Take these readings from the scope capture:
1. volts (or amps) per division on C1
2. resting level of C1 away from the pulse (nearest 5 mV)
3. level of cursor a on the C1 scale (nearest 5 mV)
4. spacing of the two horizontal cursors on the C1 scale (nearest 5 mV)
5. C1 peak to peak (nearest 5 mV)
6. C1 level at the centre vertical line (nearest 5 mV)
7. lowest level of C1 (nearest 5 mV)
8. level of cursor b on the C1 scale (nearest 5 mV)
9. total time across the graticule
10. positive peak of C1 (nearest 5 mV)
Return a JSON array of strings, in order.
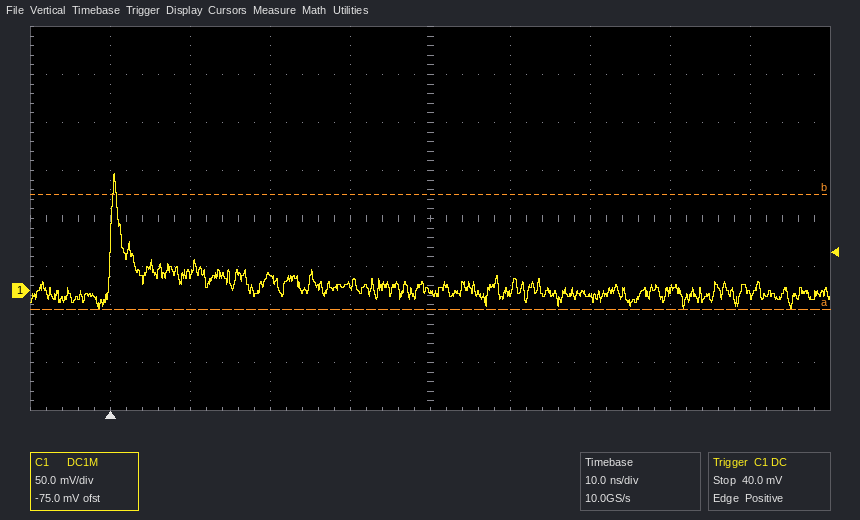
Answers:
["50 mV", "0 mV", "-20 mV", "120 mV", "140 mV", "0 mV", "-20 mV", "100 mV", "100 ns", "120 mV"]
